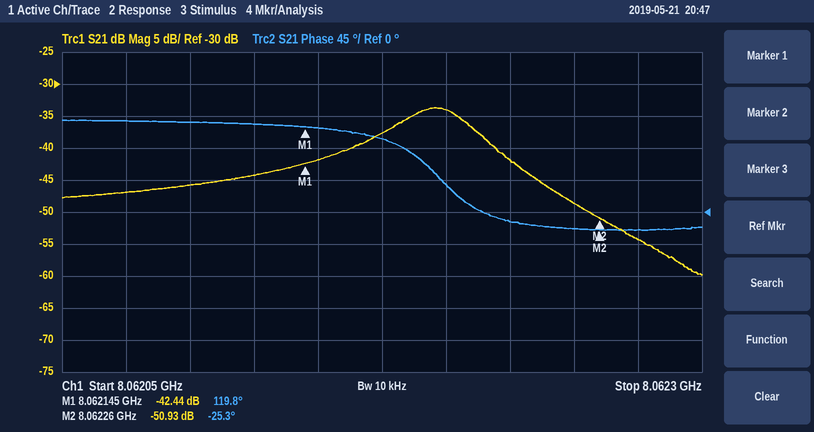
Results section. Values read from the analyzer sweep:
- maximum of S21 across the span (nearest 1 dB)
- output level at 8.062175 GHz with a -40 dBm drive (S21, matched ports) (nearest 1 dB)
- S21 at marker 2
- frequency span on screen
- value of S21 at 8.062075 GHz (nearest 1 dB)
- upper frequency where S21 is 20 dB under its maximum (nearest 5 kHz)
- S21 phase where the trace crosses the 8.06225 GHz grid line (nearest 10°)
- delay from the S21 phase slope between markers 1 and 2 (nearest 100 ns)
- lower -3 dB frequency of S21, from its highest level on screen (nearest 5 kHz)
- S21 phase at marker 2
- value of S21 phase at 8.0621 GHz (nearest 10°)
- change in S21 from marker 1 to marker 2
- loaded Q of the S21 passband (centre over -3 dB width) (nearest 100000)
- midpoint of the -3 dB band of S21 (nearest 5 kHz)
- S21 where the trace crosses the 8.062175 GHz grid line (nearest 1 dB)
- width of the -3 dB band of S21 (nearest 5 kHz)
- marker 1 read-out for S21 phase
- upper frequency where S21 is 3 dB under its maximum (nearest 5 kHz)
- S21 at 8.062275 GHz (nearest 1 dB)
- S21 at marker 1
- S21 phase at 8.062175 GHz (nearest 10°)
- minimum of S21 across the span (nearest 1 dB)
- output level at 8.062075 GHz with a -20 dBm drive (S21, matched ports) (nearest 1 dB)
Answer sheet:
-34 dB
-78 dBm
-50.93 dB
250 kHz
-47 dB
8.062270 GHz
-20°
3.5 µs
8.062180 GHz
-25.3°
130°
-8.49 dB
300000
8.062195 GHz
-38 dB
30 kHz
119.8°
8.062210 GHz
-54 dB
-42.44 dB
100°
-60 dB
-67 dBm
